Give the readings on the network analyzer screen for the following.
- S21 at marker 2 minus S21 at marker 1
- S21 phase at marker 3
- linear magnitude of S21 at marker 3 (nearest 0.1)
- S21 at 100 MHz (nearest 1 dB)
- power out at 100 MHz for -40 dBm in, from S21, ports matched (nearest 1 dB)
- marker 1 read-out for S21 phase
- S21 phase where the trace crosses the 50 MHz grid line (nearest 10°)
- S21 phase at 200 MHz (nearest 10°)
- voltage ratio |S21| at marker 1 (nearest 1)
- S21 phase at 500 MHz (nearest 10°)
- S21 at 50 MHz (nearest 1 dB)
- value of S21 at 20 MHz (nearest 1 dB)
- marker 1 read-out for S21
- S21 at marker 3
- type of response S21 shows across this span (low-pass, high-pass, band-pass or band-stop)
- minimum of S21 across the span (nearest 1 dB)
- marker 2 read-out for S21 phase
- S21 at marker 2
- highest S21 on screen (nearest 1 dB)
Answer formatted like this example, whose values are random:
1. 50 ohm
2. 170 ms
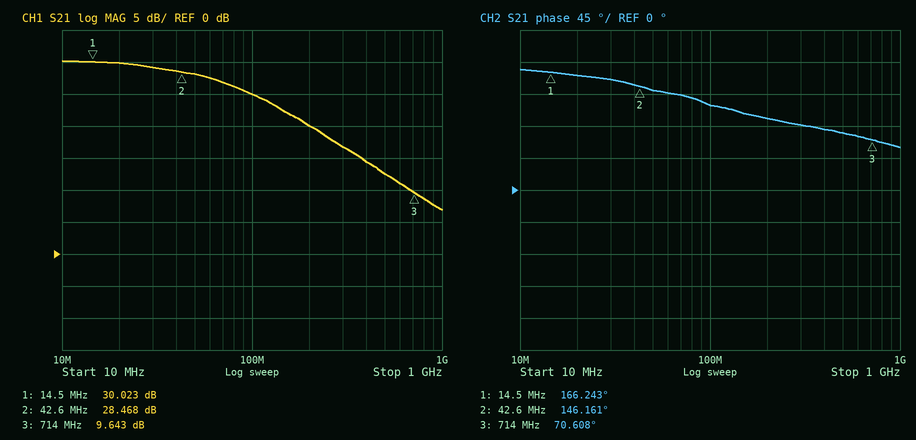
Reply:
1. -1.555 dB
2. 70.608°
3. 3.0
4. 25 dB
5. -15 dBm
6. 166.243°
7. 140°
8. 100°
9. 32
10. 80°
11. 28 dB
12. 30 dB
13. 30.023 dB
14. 9.643 dB
15. low-pass
16. 7 dB
17. 146.161°
18. 28.468 dB
19. 30 dB
